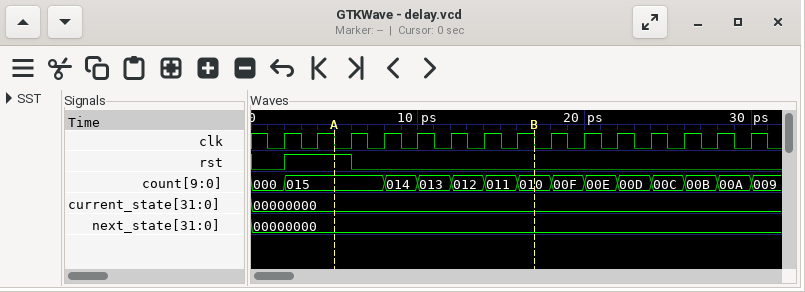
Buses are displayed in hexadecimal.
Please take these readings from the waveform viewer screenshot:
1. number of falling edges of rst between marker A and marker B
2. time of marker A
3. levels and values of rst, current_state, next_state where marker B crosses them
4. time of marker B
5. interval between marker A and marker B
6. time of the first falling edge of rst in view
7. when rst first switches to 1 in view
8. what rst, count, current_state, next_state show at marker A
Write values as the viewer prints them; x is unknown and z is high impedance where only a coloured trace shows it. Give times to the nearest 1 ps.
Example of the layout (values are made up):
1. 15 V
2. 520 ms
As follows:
1. 1
2. 5 ps
3. rst=0, current_state=00000000, next_state=00000000
4. 17 ps
5. 12 ps
6. 6 ps
7. 2 ps
8. rst=1, count=015, current_state=00000000, next_state=00000000
